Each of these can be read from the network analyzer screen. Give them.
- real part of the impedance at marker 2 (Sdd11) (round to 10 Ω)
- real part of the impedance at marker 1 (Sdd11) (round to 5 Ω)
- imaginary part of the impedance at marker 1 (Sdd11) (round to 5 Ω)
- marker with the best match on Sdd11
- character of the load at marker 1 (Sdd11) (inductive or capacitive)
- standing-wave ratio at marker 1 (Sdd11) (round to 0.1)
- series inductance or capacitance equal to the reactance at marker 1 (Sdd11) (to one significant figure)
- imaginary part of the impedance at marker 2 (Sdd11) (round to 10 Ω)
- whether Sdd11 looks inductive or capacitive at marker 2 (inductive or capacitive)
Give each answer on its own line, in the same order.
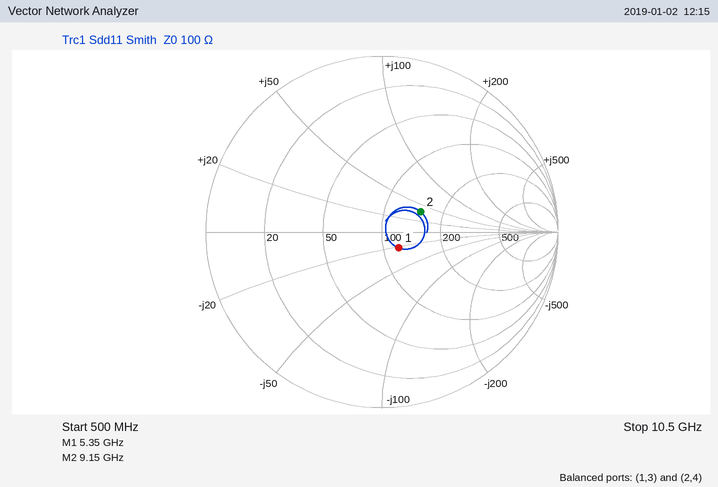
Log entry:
150 Ω
120 Ω
-20 Ω
marker 1
capacitive
1.3
1 pF
+40 Ω
inductive
